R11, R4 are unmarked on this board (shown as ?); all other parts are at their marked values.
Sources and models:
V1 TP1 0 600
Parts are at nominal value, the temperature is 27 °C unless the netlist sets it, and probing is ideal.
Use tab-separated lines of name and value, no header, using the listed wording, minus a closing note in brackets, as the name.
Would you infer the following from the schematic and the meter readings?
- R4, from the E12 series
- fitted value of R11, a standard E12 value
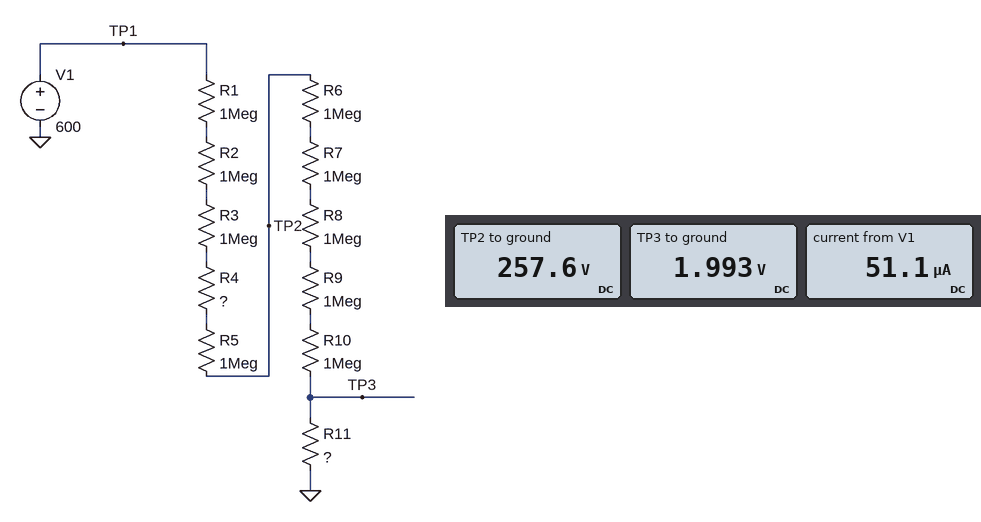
R4, from the E12 series	2.7 MΩ
fitted value of R11, a standard E12 value	39 kΩ
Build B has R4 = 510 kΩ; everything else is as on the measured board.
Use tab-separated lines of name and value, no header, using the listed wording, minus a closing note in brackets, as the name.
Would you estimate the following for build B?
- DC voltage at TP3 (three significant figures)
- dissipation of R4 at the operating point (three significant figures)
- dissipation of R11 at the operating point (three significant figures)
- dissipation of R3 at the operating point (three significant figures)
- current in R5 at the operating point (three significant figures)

DC voltage at TP3	2.45 V
dissipation of R4 at the operating point	2.01 mW
dissipation of R11 at the operating point	154 µW
dissipation of R3 at the operating point	3.95 mW
current in R5 at the operating point	62.8 µA
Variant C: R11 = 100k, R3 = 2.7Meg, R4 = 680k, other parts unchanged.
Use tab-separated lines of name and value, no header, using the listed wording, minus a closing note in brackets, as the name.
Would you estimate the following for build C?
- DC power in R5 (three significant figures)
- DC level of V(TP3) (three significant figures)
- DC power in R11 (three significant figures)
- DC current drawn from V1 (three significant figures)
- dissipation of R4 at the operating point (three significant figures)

DC power in R5	2.73 mW
DC level of V(TP3)	5.23 V
DC power in R11	273 µW
DC current drawn from V1	52.3 µA
dissipation of R4 at the operating point	1.86 mW
